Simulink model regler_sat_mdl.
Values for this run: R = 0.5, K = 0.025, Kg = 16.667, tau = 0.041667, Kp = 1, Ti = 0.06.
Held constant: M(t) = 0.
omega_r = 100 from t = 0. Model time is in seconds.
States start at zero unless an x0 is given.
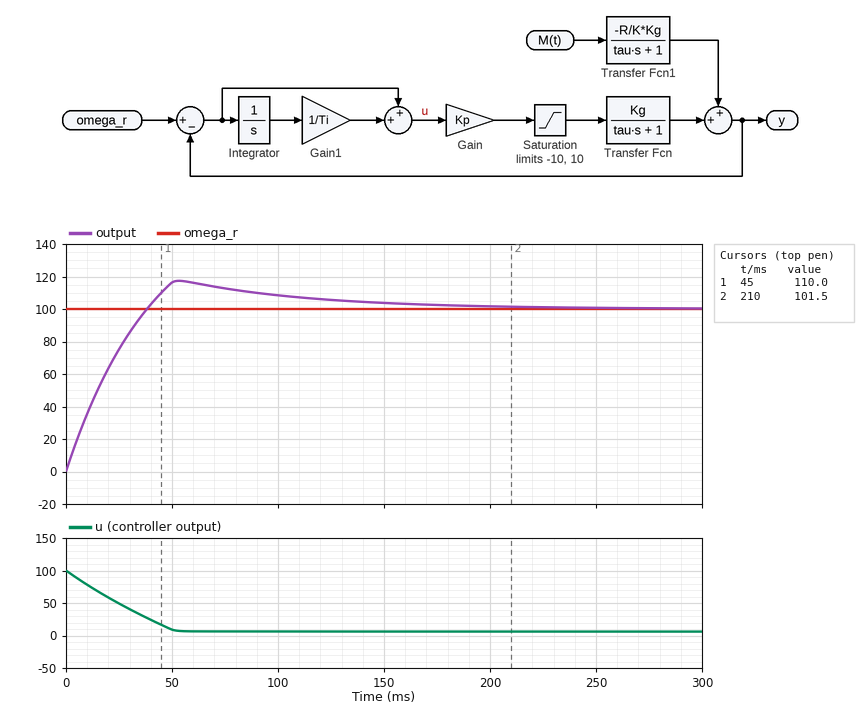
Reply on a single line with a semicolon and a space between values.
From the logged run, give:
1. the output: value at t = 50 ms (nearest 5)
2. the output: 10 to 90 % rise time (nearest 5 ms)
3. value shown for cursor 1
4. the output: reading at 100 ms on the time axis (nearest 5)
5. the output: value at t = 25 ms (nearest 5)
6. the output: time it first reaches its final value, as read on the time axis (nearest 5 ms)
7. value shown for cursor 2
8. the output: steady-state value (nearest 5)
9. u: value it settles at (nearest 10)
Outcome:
115; 30 ms; 110.0; 110; 75; 40 ms; 101.5; 100; 10
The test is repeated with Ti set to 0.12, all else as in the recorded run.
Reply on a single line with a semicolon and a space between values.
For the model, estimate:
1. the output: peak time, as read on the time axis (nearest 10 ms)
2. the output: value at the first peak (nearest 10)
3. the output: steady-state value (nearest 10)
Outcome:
50 ms; 110; 100
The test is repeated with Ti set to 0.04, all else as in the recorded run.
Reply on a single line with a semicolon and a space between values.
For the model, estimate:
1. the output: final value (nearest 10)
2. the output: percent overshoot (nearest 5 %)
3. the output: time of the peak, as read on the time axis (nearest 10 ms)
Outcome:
100; 25 %; 60 ms
